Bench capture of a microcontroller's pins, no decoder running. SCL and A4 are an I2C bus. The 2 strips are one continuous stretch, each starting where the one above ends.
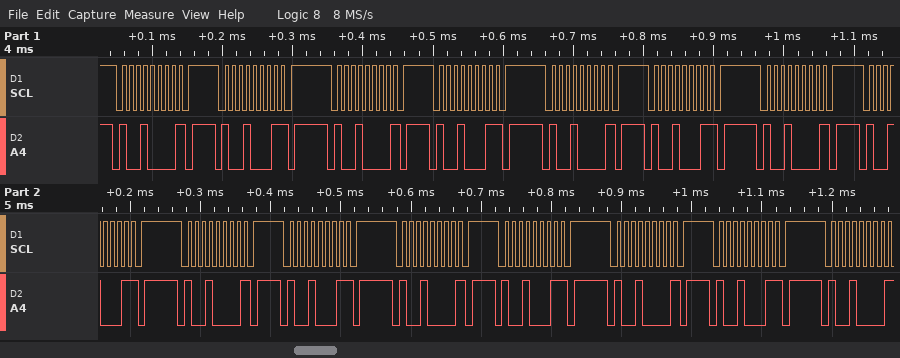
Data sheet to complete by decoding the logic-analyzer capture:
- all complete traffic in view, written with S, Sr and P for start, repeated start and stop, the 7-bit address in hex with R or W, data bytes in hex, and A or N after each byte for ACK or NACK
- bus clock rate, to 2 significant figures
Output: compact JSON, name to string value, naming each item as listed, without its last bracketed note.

{"all complete traffic in view, written with S, Sr and P for start, repeated start and stop, the 7-bit address in hex with R or W, data bytes in hex, and A or N after each byte for ACK or NACK": "S 48W N P S 48R N P S 48W N P S 48R N P S 48W N P S 48R N P S 48W N P S 48R N P S 48W N P S 48R N P S 48W N P S 48R N P S 48W N P S 48R N P S 48W N", "bus clock rate, to 2 significant figures": "100 kHz"}
